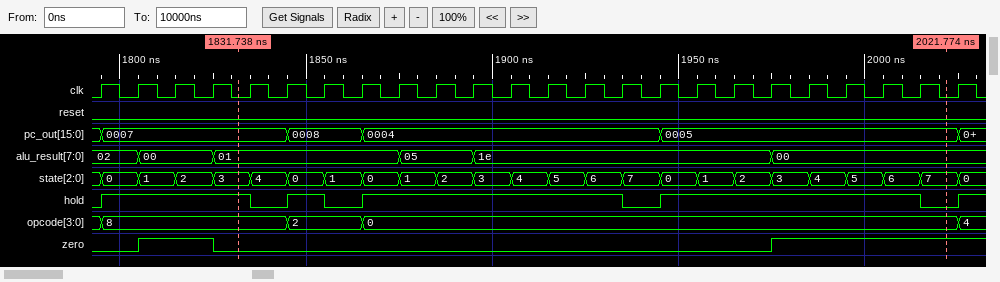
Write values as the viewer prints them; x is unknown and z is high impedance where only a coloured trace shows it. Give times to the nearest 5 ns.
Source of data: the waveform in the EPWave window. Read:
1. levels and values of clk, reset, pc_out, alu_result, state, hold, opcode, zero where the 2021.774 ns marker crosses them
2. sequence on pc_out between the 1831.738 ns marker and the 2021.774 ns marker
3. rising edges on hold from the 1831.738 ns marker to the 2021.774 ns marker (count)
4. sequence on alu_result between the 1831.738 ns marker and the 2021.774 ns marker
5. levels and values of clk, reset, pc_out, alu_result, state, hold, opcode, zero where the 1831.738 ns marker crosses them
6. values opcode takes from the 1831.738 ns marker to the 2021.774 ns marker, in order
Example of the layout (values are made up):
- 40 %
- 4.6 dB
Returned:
- clk=0, reset=0, pc_out=0005, alu_result=00, state=7, hold=0, opcode=0, zero=1
- 0007, 0008, 0004, 0005
- 3
- 01, 05, 1e, 00
- clk=0, reset=0, pc_out=0007, alu_result=01, state=3, hold=1, opcode=8, zero=0
- 8, 2, 0
